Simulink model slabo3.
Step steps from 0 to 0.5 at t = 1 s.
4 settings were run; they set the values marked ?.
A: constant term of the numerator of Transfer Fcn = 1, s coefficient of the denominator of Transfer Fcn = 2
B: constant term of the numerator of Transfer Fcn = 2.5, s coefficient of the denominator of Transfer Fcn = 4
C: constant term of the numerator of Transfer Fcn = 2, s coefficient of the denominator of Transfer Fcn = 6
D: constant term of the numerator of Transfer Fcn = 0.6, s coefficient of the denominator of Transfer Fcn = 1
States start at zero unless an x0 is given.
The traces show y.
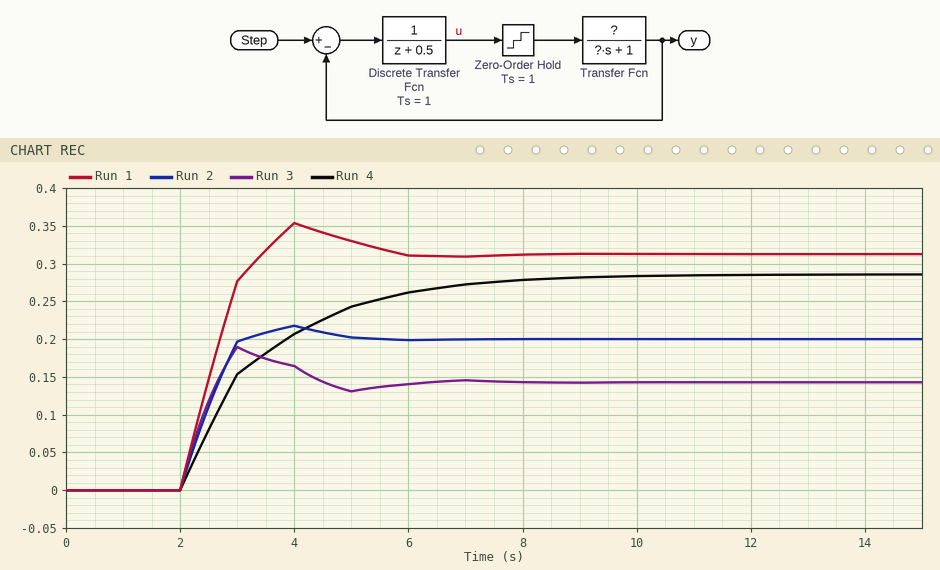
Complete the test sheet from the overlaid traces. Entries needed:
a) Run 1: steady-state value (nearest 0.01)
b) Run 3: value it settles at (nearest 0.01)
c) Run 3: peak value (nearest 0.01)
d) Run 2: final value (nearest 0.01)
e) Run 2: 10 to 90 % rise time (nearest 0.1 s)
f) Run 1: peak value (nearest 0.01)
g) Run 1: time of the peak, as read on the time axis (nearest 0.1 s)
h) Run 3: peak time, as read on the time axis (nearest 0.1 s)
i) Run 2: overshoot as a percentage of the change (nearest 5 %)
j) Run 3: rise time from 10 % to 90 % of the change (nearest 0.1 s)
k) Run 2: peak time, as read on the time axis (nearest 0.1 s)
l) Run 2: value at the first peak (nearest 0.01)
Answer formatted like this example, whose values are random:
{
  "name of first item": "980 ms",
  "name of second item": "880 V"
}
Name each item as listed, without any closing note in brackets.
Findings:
{
  "Run 1: steady-state value": "0.31",
  "Run 3: value it settles at": "0.14",
  "Run 3: peak value": "0.19",
  "Run 2: final value": "0.20",
  "Run 2: 10 to 90 % rise time": "0.8 s",
  "Run 1: peak value": "0.35",
  "Run 1: time of the peak, as read on the time axis": "4.0 s",
  "Run 3: peak time, as read on the time axis": "3.0 s",
  "Run 2: overshoot as a percentage of the change": "10 %",
  "Run 3: rise time from 10 % to 90 % of the change": "0.5 s",
  "Run 2: peak time, as read on the time axis": "4.0 s",
  "Run 2: value at the first peak": "0.22"
}
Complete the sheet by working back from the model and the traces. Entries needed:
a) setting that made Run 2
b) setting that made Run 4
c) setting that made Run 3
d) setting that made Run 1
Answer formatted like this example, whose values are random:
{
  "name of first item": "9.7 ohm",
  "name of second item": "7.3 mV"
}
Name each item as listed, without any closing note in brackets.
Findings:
{
  "setting that made Run 2": "A",
  "setting that made Run 4": "C",
  "setting that made Run 3": "D",
  "setting that made Run 1": "B"
}
